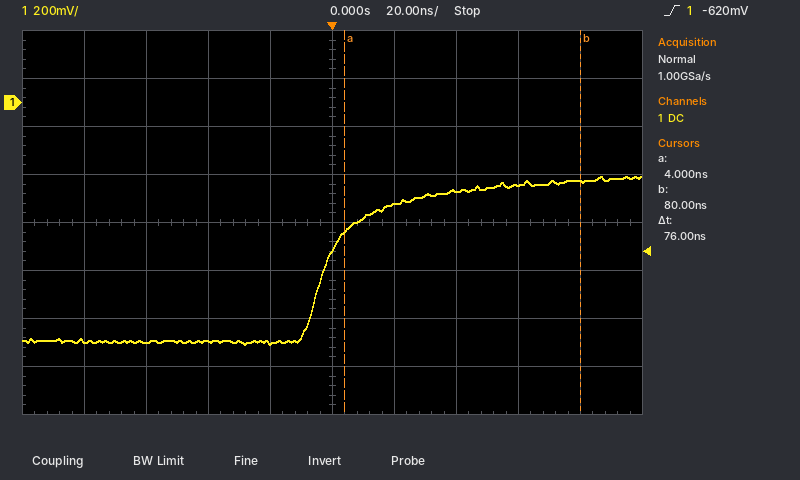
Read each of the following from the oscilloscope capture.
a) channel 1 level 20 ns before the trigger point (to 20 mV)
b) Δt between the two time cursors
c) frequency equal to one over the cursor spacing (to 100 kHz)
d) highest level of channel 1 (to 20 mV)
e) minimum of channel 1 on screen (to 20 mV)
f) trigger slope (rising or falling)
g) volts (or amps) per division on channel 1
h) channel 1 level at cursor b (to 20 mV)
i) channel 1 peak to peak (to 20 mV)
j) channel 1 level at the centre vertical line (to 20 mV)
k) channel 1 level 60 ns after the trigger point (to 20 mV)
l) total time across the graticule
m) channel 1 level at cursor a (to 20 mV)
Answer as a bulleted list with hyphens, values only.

- -1.00 V
- 76 ns
- 13.2 MHz
- -300 mV
- -1.00 V
- rising
- 200 mV
- -320 mV
- 700 mV
- -620 mV
- -340 mV
- 200 ns
- -540 mV
